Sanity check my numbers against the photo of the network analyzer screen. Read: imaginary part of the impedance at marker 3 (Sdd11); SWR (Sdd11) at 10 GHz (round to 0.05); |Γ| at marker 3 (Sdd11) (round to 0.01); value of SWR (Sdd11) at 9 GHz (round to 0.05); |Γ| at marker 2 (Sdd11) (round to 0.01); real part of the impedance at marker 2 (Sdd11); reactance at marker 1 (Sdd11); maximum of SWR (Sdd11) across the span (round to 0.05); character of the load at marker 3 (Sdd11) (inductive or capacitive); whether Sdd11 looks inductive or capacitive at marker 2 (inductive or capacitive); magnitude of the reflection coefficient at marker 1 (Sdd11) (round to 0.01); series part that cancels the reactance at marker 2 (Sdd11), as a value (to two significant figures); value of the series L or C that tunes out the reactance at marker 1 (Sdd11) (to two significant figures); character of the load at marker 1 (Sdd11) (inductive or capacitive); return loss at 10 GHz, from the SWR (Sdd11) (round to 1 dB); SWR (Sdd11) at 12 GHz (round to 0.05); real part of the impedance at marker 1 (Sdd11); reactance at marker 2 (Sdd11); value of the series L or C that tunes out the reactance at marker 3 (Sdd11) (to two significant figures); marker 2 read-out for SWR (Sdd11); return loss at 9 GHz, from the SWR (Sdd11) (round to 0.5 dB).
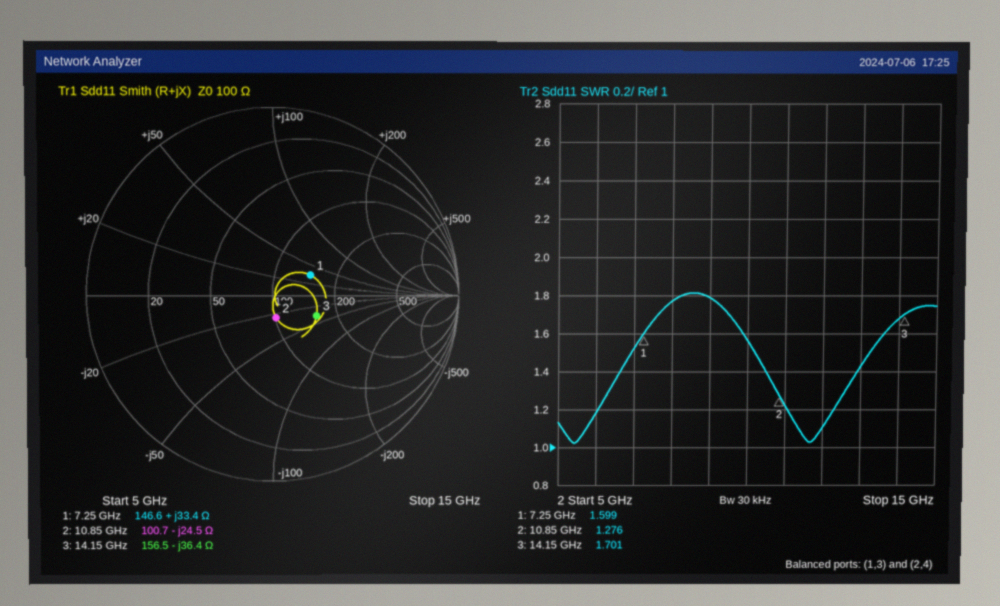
-36.4 Ω
1.55
0.26
1.80
0.12
100.7 Ω
+33.4 Ω
1.80
capacitive
capacitive
0.23
360 pH
660 fF
inductive
13 dB
1.10
146.6 Ω
-24.5 Ω
410 pH
1.276
11.0 dB
